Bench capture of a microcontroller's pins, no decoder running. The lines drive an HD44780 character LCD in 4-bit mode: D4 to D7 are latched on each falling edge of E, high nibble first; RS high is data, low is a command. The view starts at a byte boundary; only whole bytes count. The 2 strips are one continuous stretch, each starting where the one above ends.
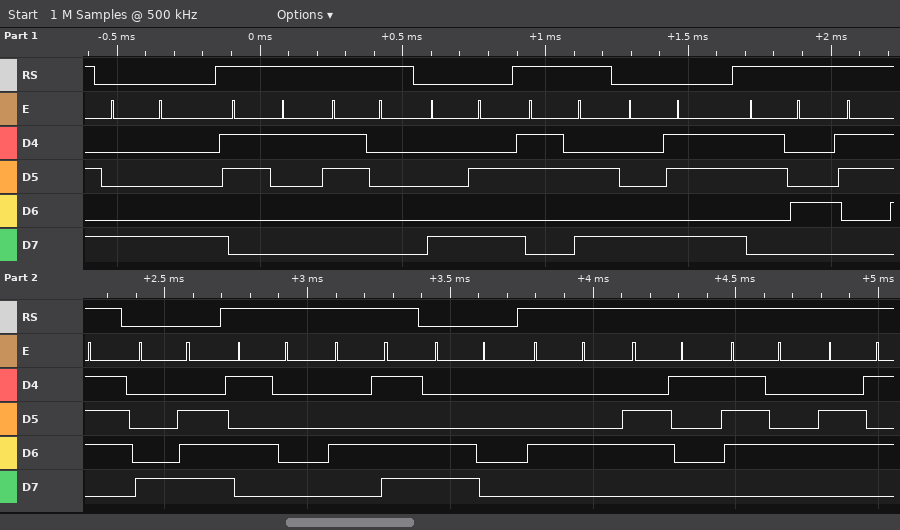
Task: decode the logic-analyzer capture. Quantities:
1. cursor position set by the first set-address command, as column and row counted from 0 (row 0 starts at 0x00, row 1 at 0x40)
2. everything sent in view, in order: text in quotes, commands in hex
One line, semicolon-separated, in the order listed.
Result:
column 8, row 0; 0x88 "10" 0x8A ":" 0x8B "47" 0x8E "PM" 0xC0 "Date"
